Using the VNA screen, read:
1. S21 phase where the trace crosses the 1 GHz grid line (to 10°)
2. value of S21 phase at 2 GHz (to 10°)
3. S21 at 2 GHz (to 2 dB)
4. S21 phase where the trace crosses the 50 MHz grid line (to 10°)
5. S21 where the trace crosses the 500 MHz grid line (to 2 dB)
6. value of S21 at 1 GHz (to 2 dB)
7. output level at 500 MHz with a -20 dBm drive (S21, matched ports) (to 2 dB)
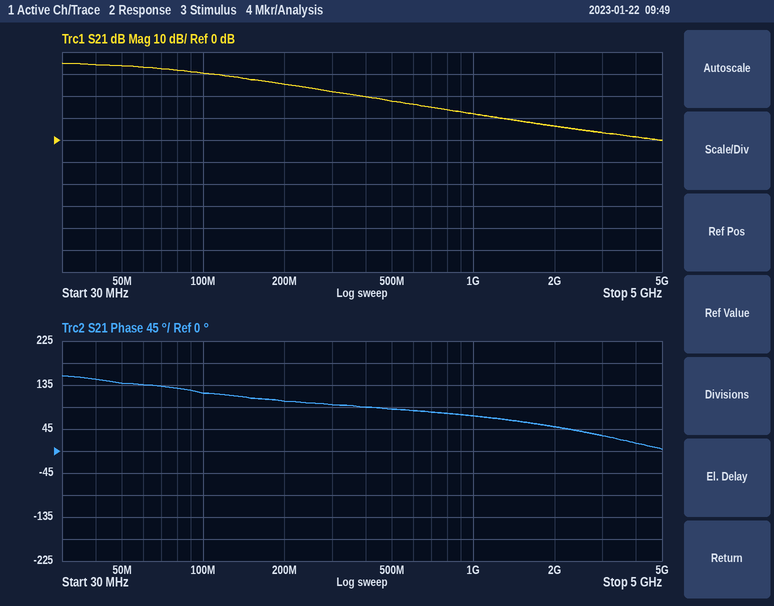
70°
50°
6 dB
140°
18 dB
12 dB
-2 dBm
